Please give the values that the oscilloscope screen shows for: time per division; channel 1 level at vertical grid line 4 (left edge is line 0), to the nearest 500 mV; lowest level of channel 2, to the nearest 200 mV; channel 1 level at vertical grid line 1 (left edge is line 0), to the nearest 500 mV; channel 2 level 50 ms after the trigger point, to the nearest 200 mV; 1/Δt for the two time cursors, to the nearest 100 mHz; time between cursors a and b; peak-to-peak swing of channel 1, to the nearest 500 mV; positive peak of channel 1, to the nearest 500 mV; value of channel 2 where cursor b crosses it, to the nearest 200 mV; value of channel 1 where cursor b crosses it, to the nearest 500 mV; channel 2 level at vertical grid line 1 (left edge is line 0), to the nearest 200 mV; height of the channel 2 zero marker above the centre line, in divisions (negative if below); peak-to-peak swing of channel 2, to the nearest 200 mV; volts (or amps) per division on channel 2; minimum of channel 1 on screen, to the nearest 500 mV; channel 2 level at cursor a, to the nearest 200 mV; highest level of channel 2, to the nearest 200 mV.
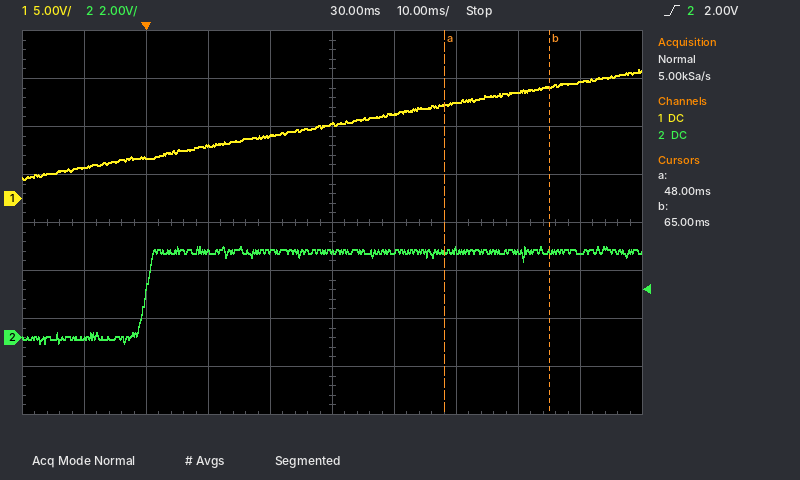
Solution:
10 ms
6.5 V
-200 mV
3.0 V
3.6 V
58.8 Hz
17 ms
11.5 V
13.5 V
3.6 V
11.5 V
0.0 V
-2.4 div
4.0 V
2 V
2.0 V
3.6 V
3.8 V
